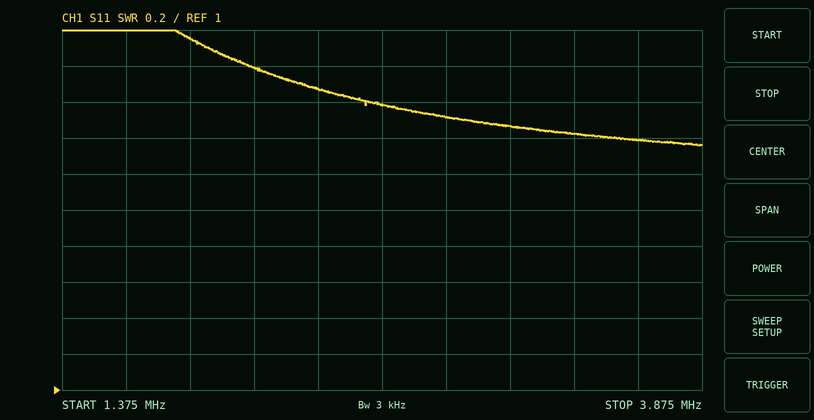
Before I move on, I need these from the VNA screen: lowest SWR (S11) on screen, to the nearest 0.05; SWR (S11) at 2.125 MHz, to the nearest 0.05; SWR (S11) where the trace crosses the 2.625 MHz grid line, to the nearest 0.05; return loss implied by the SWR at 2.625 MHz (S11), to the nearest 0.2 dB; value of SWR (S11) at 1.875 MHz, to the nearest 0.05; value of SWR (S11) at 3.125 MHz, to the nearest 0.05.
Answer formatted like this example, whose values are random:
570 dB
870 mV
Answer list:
2.35
2.80
2.60
7.0 dB
2.95
2.45
